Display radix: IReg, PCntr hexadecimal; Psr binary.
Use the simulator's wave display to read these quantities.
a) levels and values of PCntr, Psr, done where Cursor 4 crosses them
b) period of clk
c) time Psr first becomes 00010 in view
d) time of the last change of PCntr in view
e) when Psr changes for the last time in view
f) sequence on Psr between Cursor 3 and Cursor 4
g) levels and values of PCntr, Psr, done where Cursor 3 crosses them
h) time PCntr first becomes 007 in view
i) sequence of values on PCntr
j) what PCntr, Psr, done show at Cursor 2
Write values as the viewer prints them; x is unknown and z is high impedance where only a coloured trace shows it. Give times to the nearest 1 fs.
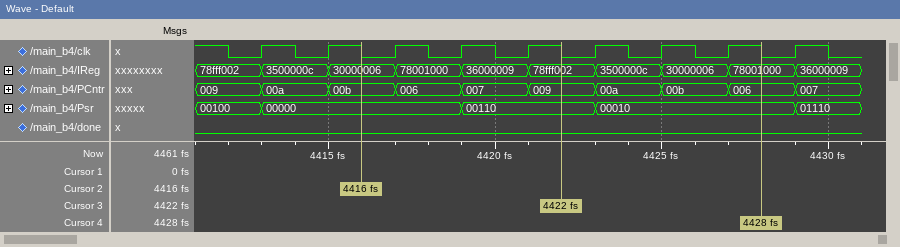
PCntr=006, Psr=00010, done=0
2 fs
4423 fs
4429 fs
4429 fs
00110, 00010
PCntr=009, Psr=00110, done=0
4419 fs
009, 00a, 00b, 006, 007, 009, 00a, 00b, 006, 007
PCntr=00b, Psr=00000, done=0
